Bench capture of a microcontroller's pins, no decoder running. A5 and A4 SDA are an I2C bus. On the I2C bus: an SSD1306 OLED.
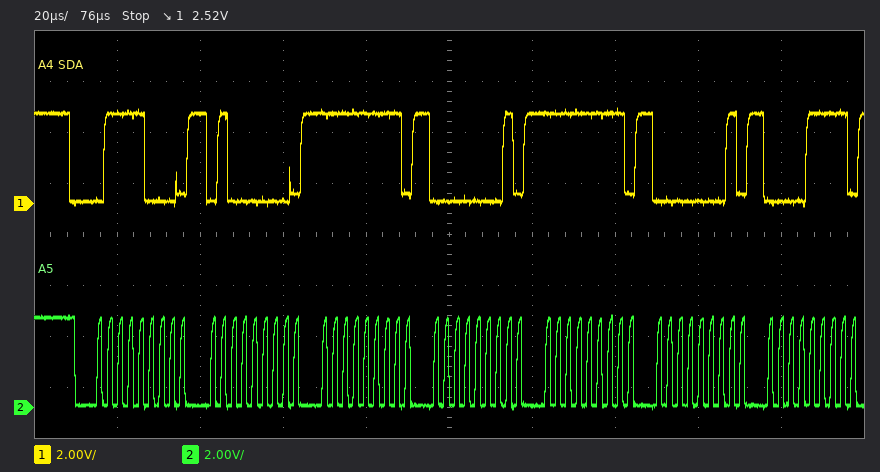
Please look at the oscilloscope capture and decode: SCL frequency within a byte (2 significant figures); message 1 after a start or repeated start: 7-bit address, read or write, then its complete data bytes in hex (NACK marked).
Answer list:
400 kHz
0x3C write: 40 FF 01 FF 01 0F
